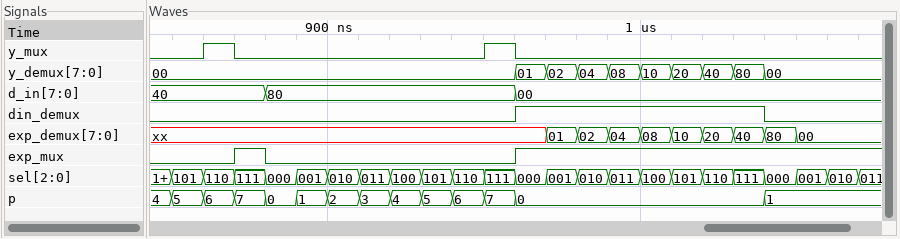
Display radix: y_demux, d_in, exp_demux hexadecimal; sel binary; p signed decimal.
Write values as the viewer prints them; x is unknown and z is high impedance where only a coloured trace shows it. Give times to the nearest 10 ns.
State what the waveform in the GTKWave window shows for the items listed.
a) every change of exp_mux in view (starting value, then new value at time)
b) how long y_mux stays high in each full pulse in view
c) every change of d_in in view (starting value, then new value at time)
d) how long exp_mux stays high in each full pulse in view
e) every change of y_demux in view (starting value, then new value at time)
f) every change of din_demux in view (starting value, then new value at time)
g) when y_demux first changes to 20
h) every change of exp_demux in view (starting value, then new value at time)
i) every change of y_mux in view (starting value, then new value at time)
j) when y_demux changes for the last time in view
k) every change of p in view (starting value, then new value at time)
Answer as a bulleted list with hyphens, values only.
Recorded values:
- 0, 1 at 870 ns, 0 at 880 ns, 1 at 960 ns
- 10 ns, 10 ns
- 40, 80 at 880 ns, 00 at 960 ns
- 10 ns
- 00, 01 at 960 ns, 02 at 970 ns, 04 at 980 ns, 08 at 990 ns, 10 at 1000 ns, 20 at 1010 ns, 40 at 1020 ns, 80 at 1030 ns, 00 at 1040 ns
- 0, 1 at 960 ns, 0 at 1040 ns
- 1010 ns
- xx, 01 at 970 ns, 02 at 980 ns, 04 at 990 ns, 08 at 1000 ns, 10 at 1010 ns, 20 at 1020 ns, 40 at 1030 ns, 80 at 1040 ns, 00 at 1050 ns
- 0, 1 at 860 ns, 0 at 870 ns, 1 at 950 ns, 0 at 960 ns
- 1040 ns
- 4, 5 at 850 ns, 6 at 860 ns, 7 at 870 ns, 0 at 880 ns, 1 at 890 ns, 2 at 900 ns, 3 at 910 ns, 4 at 920 ns, 5 at 930 ns, 6 at 940 ns, 7 at 950 ns, 0 at 960 ns, 1 at 1040 ns
